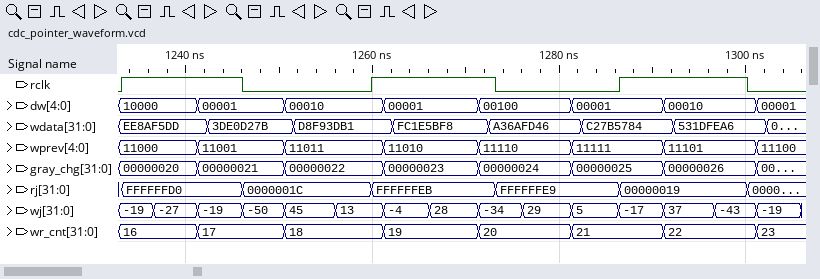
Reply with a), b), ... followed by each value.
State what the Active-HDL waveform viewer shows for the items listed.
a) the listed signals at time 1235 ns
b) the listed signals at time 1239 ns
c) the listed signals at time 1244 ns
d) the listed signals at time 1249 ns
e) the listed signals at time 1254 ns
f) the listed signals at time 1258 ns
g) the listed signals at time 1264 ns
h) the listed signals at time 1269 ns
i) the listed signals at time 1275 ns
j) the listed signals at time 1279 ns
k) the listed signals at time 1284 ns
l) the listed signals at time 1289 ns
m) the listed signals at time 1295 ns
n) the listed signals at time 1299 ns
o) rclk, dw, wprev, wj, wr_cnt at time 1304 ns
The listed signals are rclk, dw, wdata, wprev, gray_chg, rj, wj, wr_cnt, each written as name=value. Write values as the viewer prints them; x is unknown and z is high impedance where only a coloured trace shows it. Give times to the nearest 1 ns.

a) rclk=1, dw=10000, wdata=EE8AF5DD, wprev=11000, gray_chg=00000020, rj=FFFFFFD0, wj=-19, wr_cnt=16
b) rclk=1, dw=10000, wdata=EE8AF5DD, wprev=11000, gray_chg=00000020, rj=FFFFFFD0, wj=-27, wr_cnt=16
c) rclk=1, dw=00001, wdata=3DE0D27B, wprev=11001, gray_chg=00000021, rj=FFFFFFD0, wj=-19, wr_cnt=17
d) rclk=0, dw=00001, wdata=3DE0D27B, wprev=11001, gray_chg=00000021, rj=0000001C, wj=-50, wr_cnt=17
e) rclk=0, dw=00010, wdata=D8F93DB1, wprev=11011, gray_chg=00000022, rj=0000001C, wj=45, wr_cnt=18
f) rclk=0, dw=00010, wdata=D8F93DB1, wprev=11011, gray_chg=00000022, rj=0000001C, wj=13, wr_cnt=18
g) rclk=1, dw=00001, wdata=FC1E5BF8, wprev=11010, gray_chg=00000023, rj=FFFFFFEB, wj=-4, wr_cnt=19
h) rclk=1, dw=00001, wdata=FC1E5BF8, wprev=11010, gray_chg=00000023, rj=FFFFFFEB, wj=28, wr_cnt=19
i) rclk=0, dw=00100, wdata=A36AFD46, wprev=11110, gray_chg=00000024, rj=FFFFFFE9, wj=-34, wr_cnt=20
j) rclk=0, dw=00100, wdata=A36AFD46, wprev=11110, gray_chg=00000024, rj=FFFFFFE9, wj=29, wr_cnt=20
k) rclk=0, dw=00001, wdata=C27B5784, wprev=11111, gray_chg=00000025, rj=FFFFFFE9, wj=5, wr_cnt=21
l) rclk=1, dw=00001, wdata=C27B5784, wprev=11111, gray_chg=00000025, rj=00000019, wj=-17, wr_cnt=21
m) rclk=1, dw=00010, wdata=531DFEA6, wprev=11101, gray_chg=00000026, rj=00000019, wj=37, wr_cnt=22
n) rclk=1, dw=00010, wdata=531DFEA6, wprev=11101, gray_chg=00000026, rj=00000019, wj=-43, wr_cnt=22
o) rclk=0, dw=00001, wprev=11100, wj=-19, wr_cnt=23
